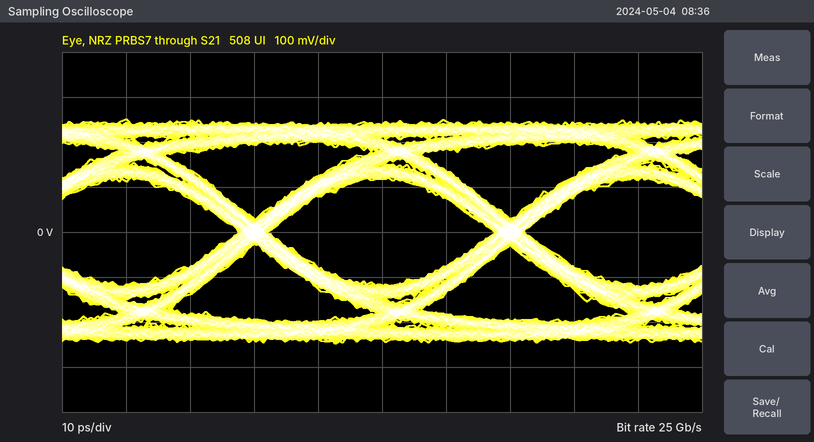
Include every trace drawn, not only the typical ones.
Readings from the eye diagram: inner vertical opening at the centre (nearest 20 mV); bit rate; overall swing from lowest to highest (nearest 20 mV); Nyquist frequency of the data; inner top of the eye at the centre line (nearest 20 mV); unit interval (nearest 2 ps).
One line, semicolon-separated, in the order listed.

240 mV; 25 Gb/s; 500 mV; 12.5 GHz; 120 mV; 40 ps
